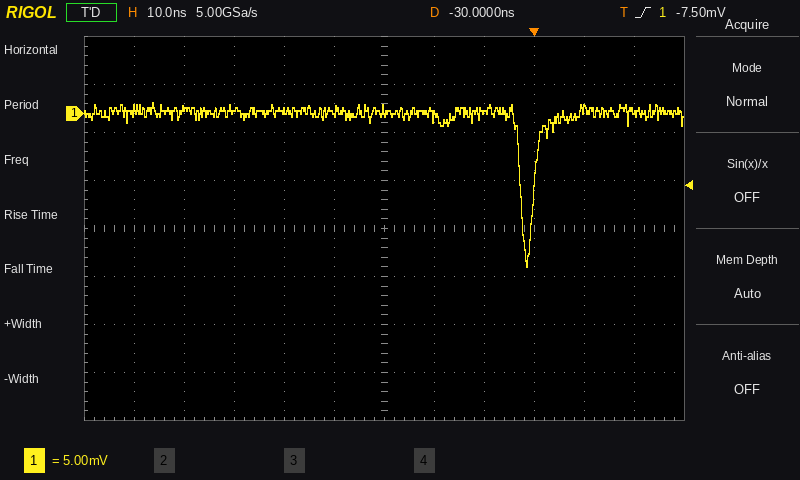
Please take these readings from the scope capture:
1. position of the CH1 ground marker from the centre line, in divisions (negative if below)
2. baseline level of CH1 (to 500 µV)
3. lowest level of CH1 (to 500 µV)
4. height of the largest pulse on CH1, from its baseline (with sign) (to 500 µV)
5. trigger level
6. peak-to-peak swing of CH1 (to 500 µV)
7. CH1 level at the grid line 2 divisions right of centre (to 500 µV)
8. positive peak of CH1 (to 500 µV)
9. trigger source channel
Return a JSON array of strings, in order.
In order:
["+2.4 div", "0.0 mV", "-16.0 mV", "-16.0 mV", "-7.50 mV", "17.0 mV", "0.0 mV", "1.0 mV", "CH1"]
